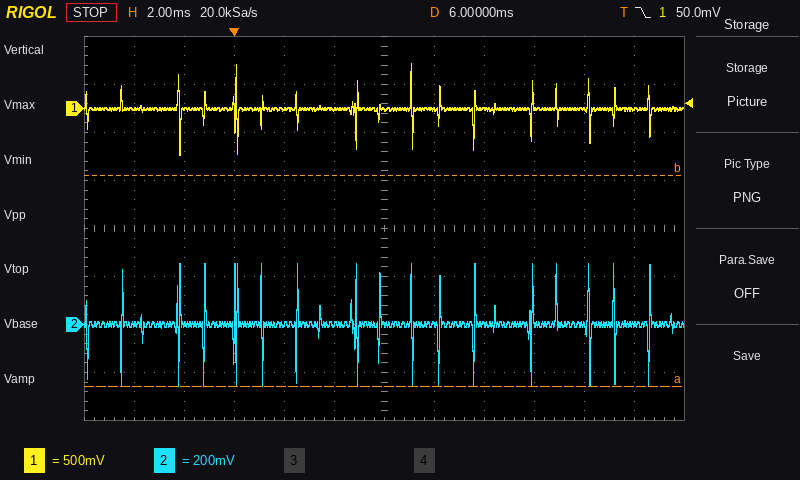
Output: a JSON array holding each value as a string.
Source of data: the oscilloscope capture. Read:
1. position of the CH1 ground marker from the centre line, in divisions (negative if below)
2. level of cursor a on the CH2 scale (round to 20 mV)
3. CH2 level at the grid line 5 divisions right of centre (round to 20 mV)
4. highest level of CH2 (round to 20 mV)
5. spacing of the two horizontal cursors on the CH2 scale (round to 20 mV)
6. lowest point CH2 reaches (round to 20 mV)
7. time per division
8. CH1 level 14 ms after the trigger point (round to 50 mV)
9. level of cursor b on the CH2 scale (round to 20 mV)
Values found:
["+2.5 div", "-260 mV", "0 mV", "260 mV", "880 mV", "-260 mV", "2 ms", "0 mV", "620 mV"]
